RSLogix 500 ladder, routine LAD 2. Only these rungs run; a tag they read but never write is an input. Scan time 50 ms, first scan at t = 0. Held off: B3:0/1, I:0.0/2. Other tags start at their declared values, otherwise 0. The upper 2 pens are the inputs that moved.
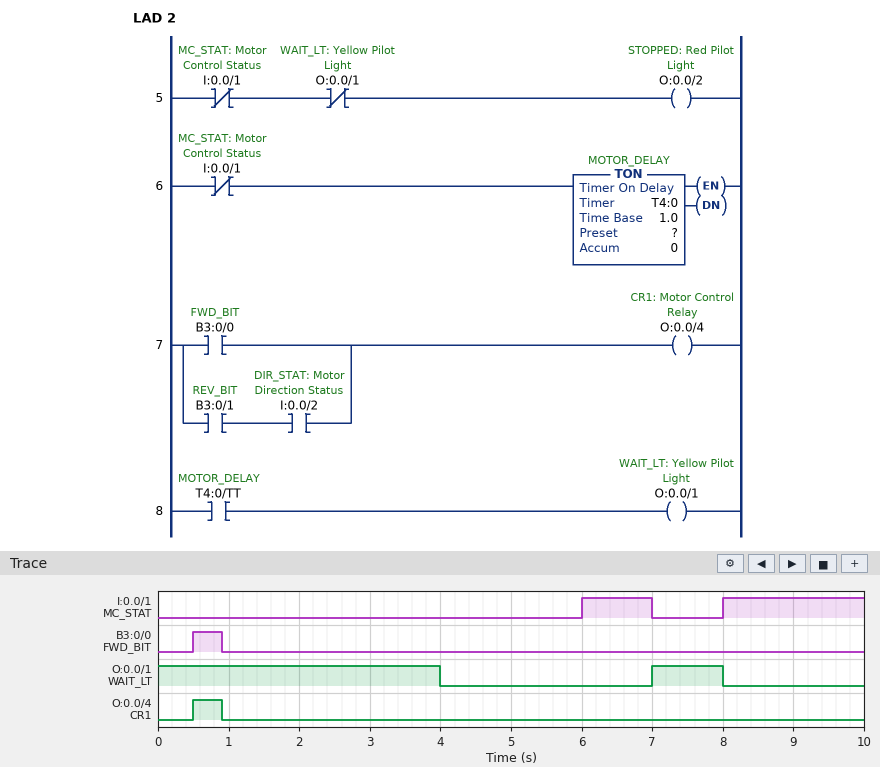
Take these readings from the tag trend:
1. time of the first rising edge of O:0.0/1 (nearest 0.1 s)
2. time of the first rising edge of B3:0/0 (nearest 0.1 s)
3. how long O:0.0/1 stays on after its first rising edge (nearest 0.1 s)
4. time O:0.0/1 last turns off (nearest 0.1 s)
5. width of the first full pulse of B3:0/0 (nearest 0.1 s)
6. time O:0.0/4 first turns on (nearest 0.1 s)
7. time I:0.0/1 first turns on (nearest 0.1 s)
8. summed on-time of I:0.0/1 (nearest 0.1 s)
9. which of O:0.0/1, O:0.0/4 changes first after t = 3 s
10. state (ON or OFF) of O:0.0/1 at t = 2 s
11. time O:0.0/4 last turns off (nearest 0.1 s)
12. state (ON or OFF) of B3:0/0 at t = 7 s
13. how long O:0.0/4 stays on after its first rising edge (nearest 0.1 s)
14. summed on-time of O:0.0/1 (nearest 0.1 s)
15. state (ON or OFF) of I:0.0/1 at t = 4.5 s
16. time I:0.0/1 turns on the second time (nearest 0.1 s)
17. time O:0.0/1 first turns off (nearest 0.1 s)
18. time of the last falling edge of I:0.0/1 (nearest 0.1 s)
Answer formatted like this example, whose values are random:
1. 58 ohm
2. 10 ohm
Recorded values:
1. 7.0 s
2. 0.5 s
3. 1.0 s
4. 8.0 s
5. 0.4 s
6. 0.5 s
7. 6.0 s
8. 3.0 s
9. O:0.0/1
10. ON
11. 0.9 s
12. OFF
13. 0.4 s
14. 5.0 s
15. OFF
16. 8.0 s
17. 4.0 s
18. 7.0 s
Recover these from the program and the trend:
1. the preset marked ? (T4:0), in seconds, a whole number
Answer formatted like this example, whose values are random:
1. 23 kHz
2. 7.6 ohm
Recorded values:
1. 4 s
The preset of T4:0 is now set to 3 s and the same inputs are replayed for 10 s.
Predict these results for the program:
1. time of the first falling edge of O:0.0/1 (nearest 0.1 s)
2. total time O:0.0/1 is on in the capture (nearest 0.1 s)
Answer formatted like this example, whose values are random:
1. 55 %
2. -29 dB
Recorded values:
1. 3.0 s
2. 4.0 s
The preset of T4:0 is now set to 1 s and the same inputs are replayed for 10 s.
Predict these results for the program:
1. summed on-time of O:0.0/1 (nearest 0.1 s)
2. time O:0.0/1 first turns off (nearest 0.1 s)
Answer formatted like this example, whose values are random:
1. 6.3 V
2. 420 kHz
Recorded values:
1. 2.0 s
2. 1.0 s
